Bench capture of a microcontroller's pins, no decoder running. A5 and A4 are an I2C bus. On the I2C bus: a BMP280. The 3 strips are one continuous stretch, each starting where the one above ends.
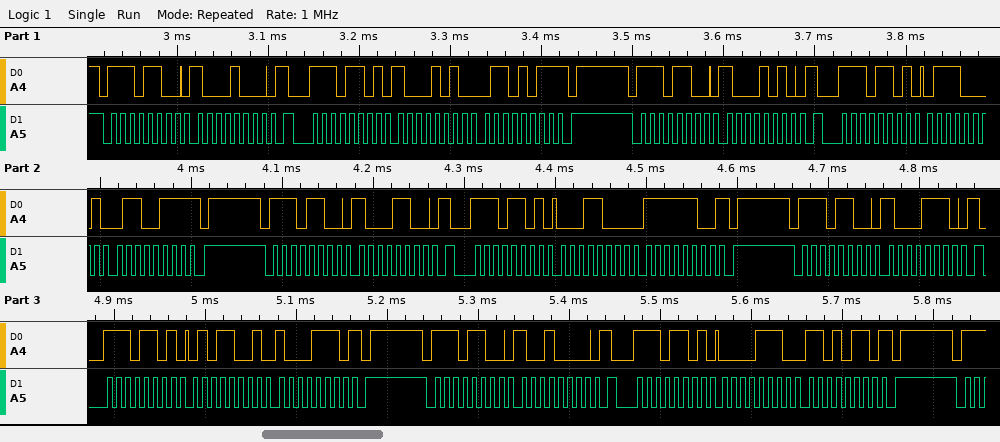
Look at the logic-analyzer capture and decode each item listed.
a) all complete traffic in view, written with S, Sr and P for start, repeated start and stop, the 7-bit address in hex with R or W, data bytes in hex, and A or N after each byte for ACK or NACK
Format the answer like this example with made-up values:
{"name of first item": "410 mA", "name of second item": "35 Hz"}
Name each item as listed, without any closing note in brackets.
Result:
{"all complete traffic in view, written with S, Sr and P for start, repeated start and stop, the 7-bit address in hex with R or W, data bytes in hex, and A or N after each byte for ACK or NACK": "S 76W A 88 A Sr 76R A 8A A 6B N P S 76W A 8A A Sr 76R A 71 A 67 N P S 76W A 8C A Sr 76R A 18 A FC N P S 76W A 8E A Sr 76R A 59 A 8E N P S 76W A 90 A Sr 76R A 0E A D6 N P"}
